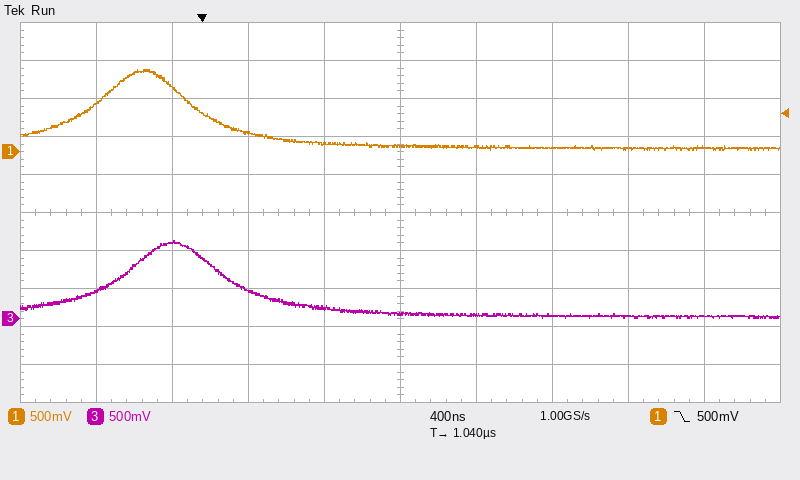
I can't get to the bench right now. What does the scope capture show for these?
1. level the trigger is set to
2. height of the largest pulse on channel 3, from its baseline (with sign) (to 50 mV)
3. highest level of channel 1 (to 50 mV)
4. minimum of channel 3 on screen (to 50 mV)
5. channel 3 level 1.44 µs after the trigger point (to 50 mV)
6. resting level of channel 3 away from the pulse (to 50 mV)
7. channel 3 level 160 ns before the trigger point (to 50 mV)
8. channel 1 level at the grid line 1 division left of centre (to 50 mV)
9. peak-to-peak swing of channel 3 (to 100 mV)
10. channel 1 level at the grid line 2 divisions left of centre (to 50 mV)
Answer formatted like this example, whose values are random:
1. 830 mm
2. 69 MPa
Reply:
1. 500 mV
2. +1.00 V
3. 1.10 V
4. 0 mV
5. 50 mV
6. 50 mV
7. 1.00 V
8. 100 mV
9. 1.00 V
10. 250 mV
